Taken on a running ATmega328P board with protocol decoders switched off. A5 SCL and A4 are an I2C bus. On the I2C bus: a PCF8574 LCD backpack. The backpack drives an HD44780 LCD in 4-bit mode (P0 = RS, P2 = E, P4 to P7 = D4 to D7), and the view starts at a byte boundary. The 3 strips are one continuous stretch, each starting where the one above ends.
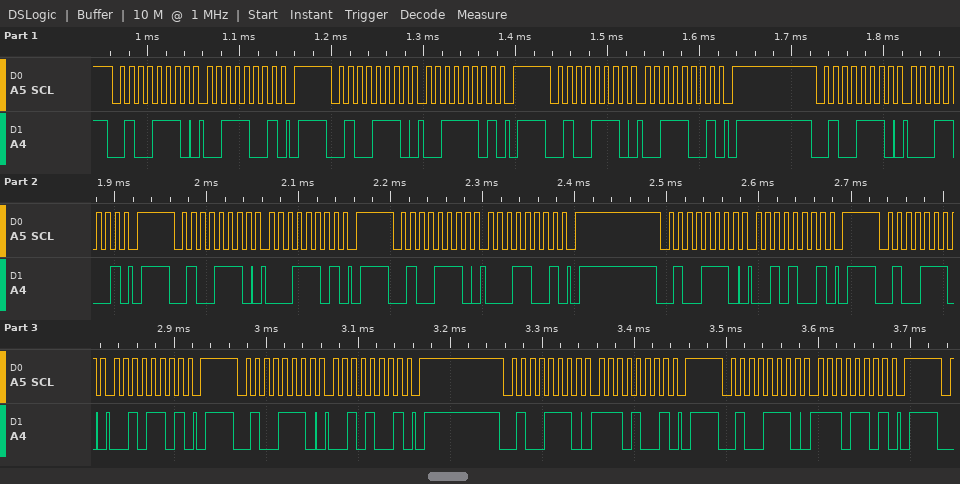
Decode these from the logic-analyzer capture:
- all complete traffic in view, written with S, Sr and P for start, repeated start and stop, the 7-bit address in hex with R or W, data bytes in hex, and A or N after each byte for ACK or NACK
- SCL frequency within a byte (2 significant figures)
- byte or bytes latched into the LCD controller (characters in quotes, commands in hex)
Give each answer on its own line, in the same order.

S 27W A 39 A P S 27W A 3D A P S 27W A 39 A P S 27W A 19 A P S 27W A 1D A P S 27W A 19 A P S 27W A 29 A P S 27W A 2D A P S 27W A 29 A P S 27W A E9 A P S 27W A ED A P
100 kHz
'1'
